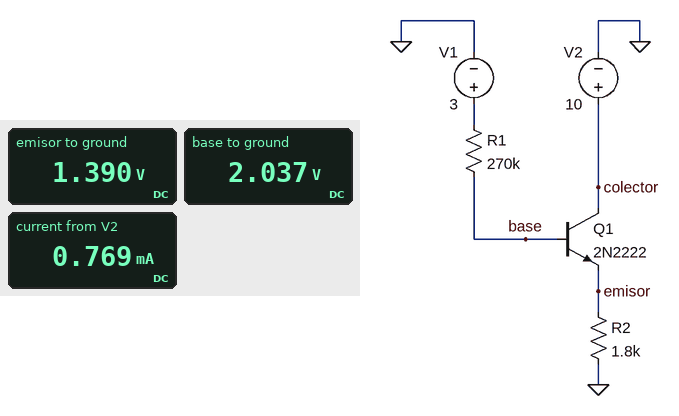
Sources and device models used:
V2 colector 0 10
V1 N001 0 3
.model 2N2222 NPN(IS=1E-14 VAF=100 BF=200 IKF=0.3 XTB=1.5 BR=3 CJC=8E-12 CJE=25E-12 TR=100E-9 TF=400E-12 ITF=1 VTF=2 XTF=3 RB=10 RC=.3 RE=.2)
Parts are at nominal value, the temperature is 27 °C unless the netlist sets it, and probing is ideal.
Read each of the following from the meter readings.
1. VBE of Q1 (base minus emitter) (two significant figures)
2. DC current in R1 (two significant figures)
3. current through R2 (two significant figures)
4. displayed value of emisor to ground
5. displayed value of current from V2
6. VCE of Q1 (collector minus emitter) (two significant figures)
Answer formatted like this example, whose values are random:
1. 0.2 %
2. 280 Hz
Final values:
1. 650 mV
2. 3.6 µA
3. 770 µA
4. 1.390 V
5. 0.769 mA
6. 8.6 V
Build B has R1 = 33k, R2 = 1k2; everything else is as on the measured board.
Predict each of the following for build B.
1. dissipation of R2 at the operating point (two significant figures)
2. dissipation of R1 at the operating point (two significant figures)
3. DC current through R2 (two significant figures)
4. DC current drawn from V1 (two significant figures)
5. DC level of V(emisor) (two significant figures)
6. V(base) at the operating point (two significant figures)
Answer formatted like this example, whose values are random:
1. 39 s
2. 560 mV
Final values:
1. 3.6 mW
2. 2.1 µW
3. 1.7 mA
4. 8.0 µA
5. 2.1 V
6. 2.7 V
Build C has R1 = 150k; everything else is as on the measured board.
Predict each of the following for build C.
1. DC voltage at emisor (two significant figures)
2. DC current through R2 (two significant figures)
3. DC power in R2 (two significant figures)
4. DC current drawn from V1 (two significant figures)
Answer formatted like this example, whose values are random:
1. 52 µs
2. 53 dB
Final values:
1. 1.7 V
2. 940 µA
3. 1.6 mW
4. 4.4 µA
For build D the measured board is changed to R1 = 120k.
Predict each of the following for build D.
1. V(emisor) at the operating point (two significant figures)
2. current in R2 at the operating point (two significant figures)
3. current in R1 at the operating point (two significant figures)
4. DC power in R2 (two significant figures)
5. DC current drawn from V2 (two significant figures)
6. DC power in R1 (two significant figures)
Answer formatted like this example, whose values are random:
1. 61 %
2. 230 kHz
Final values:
1. 1.8 V
2. 1.0 mA
3. 4.6 µA
4. 1.8 mW
5. 990 µA
6. 2.6 µW
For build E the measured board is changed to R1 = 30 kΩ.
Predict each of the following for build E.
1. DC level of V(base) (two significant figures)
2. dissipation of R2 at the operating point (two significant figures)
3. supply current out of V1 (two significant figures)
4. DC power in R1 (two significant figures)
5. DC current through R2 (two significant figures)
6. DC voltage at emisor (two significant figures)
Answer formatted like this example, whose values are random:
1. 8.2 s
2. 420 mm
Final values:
1. 2.8 V
2. 2.6 mW
3. 5.6 µA
4. 950 nW
5. 1.2 mA
6. 2.2 V
